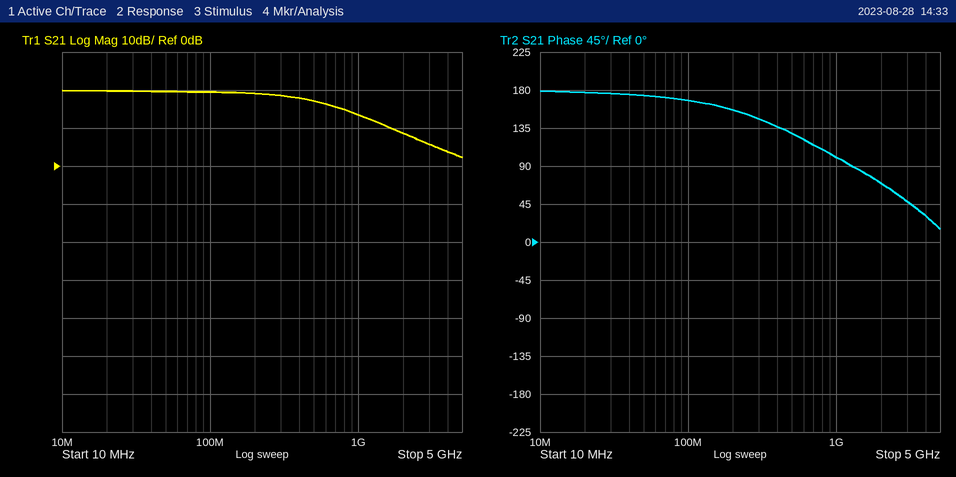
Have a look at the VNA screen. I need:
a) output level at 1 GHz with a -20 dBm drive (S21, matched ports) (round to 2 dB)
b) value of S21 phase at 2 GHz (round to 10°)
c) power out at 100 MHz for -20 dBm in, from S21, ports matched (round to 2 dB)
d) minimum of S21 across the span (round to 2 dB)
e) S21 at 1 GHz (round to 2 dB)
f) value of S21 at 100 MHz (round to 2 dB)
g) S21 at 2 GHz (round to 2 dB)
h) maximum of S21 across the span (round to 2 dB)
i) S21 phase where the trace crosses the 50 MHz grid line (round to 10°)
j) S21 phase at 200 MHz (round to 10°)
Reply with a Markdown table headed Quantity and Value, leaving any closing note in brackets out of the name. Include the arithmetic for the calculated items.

| Quantity | Value |
|---|---|
| output level at 1 GHz with a -20 dBm drive (S21, matched ports) | -20 dBm + (14 dB) = -6 dBm |
| value of S21 phase at 2 GHz | 70° |
| power out at 100 MHz for -20 dBm in, from S21, ports matched | -20 dBm + (20 dB) = 0 dBm |
| minimum of S21 across the span | 2 dB |
| S21 at 1 GHz | 14 dB |
| value of S21 at 100 MHz | 20 dB |
| S21 at 2 GHz | 8 dB |
| maximum of S21 across the span | 20 dB |
| S21 phase where the trace crosses the 50 MHz grid line | 170° |
| S21 phase at 200 MHz | 160° |
